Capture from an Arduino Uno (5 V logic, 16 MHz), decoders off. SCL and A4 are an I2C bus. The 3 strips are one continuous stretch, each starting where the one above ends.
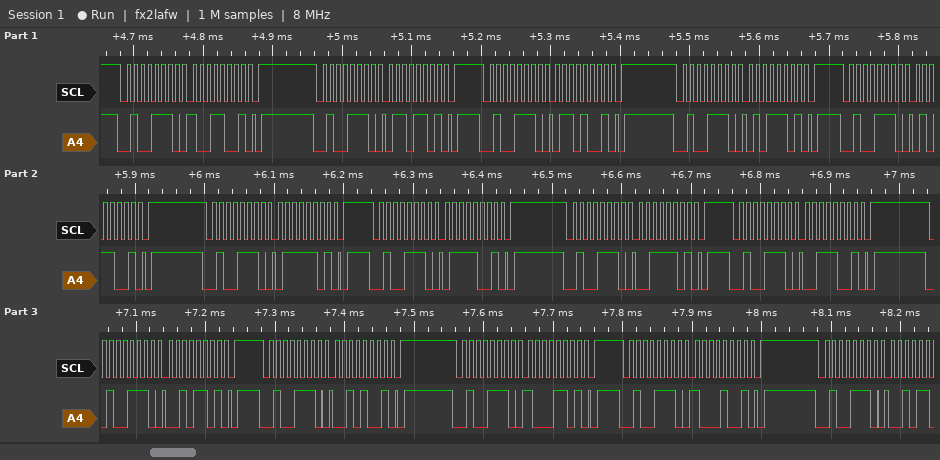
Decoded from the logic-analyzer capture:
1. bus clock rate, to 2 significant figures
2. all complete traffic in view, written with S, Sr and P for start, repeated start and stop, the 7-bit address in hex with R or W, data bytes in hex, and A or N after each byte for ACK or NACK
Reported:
100 kHz
S 27W A 99 A P S 27W A 6D A P S 27W A 69 A P S 27W A 5D A P S 27W A 59 A P S 27W A 7D A P S 27W A 79 A P S 27W A 3D A P S 27W A 39 A P S 27W A 2D A P S 27W A 29 A P S 27W A 8D A P S 27W A 89 A P S 27W A
